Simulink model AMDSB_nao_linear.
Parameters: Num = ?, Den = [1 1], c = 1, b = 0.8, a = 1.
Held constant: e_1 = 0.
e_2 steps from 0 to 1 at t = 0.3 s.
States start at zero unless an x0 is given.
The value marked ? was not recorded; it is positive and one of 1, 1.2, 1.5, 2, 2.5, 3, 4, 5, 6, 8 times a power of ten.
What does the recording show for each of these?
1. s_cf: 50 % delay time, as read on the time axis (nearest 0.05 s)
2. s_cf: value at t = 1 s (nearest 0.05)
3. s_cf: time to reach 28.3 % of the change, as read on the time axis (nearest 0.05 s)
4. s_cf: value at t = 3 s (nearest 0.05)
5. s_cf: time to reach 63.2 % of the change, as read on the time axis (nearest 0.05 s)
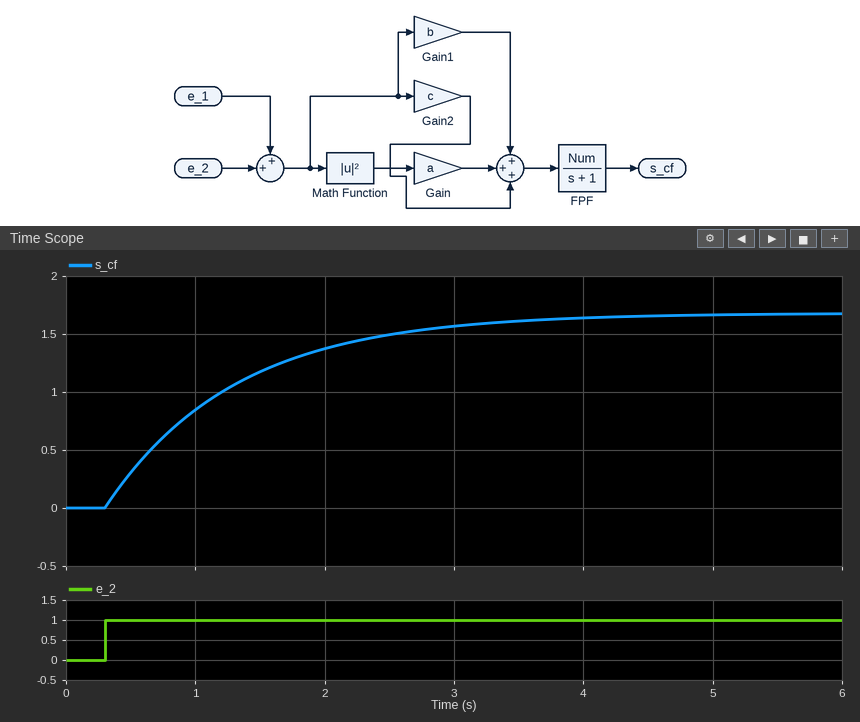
1.00 s
0.85
0.65 s
1.55
1.30 s
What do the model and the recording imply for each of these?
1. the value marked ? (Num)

0.6
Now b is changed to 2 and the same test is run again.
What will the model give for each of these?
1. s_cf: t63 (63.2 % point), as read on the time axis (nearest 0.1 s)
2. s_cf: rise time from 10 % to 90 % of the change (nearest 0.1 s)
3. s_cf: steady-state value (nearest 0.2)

1.3 s
2.2 s
2.4
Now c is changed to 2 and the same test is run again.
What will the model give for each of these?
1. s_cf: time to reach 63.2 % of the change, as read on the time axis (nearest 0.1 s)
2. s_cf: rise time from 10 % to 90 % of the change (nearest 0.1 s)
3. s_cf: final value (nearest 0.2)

1.3 s
2.2 s
2.2
